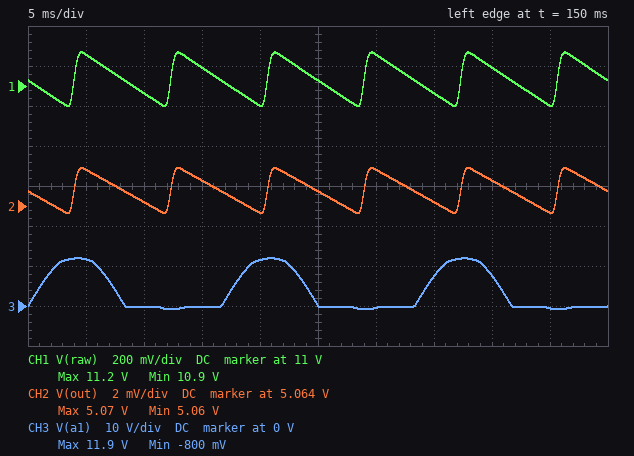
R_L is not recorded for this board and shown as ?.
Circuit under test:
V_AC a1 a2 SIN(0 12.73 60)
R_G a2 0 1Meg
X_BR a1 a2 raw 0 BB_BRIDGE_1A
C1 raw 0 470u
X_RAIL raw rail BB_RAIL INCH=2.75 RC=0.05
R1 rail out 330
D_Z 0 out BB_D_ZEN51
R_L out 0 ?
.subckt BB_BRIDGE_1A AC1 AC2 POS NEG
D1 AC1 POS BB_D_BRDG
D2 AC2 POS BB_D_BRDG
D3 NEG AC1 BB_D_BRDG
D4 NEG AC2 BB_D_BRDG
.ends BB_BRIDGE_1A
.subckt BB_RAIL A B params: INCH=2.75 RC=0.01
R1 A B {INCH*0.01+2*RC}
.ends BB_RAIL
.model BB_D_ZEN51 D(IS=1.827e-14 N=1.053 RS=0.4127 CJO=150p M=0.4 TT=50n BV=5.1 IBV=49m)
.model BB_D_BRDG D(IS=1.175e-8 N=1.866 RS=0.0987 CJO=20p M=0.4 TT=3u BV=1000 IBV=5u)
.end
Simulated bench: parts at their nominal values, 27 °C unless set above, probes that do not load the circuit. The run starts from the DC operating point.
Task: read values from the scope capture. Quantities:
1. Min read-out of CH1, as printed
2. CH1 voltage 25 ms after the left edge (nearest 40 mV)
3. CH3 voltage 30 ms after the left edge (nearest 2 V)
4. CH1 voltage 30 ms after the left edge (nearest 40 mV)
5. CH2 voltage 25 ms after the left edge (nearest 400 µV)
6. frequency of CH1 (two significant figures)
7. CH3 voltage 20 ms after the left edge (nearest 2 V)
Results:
10.9 V
11.04 V
0 V
11.16 V
5.0648 V
120 Hz
12 V
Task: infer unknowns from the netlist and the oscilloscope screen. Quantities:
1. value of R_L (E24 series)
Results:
750 Ω
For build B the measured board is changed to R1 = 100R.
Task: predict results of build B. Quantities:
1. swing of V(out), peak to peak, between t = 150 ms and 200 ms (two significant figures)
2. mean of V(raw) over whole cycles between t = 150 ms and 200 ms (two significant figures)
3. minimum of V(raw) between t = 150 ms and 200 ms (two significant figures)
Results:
7.7 mV
11 V
10 V
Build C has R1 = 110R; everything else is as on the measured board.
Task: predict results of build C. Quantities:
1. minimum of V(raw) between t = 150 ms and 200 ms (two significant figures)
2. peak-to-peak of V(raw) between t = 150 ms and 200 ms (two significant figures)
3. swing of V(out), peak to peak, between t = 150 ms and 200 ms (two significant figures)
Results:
10 V
740 mV
6.8 mV
